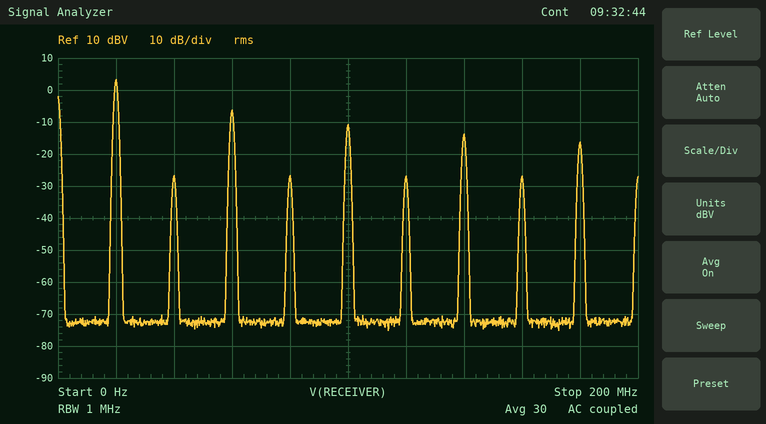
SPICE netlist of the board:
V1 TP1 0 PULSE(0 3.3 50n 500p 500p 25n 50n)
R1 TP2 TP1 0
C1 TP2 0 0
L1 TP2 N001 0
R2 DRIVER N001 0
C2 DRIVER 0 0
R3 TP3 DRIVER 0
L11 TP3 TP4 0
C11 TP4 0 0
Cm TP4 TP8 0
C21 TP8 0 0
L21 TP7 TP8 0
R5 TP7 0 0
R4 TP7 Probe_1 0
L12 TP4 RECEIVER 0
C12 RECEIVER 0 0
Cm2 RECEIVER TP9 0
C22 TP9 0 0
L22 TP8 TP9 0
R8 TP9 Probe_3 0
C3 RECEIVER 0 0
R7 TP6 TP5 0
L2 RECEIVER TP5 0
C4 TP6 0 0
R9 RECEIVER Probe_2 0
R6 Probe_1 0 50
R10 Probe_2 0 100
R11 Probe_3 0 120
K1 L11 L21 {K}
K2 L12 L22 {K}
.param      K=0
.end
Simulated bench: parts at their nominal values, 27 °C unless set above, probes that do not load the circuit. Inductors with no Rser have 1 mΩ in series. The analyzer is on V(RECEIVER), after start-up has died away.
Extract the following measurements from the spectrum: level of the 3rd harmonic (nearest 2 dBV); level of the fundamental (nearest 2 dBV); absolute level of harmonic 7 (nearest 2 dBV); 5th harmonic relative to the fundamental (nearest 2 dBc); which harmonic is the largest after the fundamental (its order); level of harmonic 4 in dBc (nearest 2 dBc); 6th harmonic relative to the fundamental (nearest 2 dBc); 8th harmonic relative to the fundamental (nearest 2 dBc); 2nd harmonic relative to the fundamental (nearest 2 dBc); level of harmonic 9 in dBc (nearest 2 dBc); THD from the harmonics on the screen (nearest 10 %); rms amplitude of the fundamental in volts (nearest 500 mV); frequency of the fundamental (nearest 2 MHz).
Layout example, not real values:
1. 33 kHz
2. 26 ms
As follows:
1. -6 dBV
2. 4 dBV
3. -14 dBV
4. -14 dBc
5. 3
6. -30 dBc
7. -30 dBc
8. -30 dBc
9. -30 dBc
10. -20 dBc
11. 40 %
12. 1.5 V
13. 20 MHz
